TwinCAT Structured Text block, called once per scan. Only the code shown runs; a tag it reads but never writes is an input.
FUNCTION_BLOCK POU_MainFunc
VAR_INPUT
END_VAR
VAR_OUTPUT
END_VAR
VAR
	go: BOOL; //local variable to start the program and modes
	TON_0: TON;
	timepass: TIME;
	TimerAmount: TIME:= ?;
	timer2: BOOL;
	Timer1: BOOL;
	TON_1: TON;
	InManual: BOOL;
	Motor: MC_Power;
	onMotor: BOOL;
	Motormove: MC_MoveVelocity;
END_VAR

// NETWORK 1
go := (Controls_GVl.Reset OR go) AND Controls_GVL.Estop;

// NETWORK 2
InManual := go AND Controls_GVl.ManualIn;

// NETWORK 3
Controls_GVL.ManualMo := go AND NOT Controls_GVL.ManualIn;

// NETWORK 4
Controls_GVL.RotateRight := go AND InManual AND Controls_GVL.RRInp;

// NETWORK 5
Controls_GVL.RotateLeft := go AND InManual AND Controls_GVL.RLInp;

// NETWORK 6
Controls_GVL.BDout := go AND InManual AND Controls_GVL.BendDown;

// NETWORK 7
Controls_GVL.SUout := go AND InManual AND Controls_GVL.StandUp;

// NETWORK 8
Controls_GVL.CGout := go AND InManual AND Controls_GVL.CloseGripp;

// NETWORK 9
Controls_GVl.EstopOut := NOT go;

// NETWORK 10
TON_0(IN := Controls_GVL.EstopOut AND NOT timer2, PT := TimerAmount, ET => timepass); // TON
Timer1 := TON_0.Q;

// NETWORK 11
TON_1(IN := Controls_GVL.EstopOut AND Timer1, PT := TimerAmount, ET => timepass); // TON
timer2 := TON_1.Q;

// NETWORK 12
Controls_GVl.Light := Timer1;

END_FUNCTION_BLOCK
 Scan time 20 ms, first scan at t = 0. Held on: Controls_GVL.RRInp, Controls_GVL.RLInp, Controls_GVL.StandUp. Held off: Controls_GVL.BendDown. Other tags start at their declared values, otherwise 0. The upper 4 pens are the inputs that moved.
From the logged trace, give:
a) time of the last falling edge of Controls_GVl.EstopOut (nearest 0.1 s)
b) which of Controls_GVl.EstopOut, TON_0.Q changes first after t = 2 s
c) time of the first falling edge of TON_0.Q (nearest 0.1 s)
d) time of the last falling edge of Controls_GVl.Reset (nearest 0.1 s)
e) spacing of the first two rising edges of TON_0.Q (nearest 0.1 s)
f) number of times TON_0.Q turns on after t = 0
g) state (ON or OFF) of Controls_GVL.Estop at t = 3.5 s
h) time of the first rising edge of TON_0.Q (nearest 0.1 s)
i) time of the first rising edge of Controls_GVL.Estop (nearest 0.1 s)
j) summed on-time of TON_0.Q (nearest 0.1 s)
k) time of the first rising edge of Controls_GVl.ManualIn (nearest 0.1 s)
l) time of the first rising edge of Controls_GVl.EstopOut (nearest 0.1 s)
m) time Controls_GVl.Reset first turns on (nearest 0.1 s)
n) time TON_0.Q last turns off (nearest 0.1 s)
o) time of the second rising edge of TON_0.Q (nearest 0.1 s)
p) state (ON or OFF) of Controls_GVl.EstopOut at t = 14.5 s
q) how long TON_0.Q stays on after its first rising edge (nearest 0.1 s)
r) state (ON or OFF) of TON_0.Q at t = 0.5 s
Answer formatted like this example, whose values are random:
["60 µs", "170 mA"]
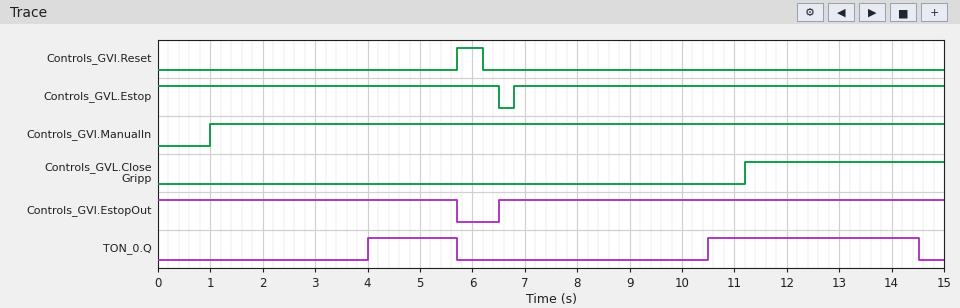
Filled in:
["5.7 s", "TON_0.Q", "5.7 s", "6.2 s", "6.5 s", "2", "ON", "4.0 s", "6.8 s", "5.7 s", "1.0 s", "6.5 s", "5.7 s", "14.5 s", "10.5 s", "ON", "1.7 s", "OFF"]
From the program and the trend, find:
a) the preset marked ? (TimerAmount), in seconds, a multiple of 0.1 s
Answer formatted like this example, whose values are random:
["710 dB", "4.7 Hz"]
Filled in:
["4.0 s"]
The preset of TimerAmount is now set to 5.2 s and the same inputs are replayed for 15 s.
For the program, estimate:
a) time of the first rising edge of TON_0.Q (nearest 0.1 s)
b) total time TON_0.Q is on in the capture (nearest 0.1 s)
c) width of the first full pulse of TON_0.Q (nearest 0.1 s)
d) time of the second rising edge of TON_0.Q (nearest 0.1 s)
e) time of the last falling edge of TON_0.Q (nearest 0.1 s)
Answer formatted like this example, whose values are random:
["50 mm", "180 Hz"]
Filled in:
["5.2 s", "3.8 s", "0.5 s", "11.7 s", "5.7 s"]
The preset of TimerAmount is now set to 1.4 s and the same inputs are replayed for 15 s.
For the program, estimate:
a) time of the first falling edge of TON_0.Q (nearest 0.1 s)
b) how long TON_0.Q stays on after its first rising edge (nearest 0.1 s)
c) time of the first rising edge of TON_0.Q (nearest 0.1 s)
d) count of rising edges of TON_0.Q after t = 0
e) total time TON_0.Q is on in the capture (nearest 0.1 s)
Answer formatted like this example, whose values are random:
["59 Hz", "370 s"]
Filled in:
["2.8 s", "1.4 s", "1.4 s", "5", "7.1 s"]
